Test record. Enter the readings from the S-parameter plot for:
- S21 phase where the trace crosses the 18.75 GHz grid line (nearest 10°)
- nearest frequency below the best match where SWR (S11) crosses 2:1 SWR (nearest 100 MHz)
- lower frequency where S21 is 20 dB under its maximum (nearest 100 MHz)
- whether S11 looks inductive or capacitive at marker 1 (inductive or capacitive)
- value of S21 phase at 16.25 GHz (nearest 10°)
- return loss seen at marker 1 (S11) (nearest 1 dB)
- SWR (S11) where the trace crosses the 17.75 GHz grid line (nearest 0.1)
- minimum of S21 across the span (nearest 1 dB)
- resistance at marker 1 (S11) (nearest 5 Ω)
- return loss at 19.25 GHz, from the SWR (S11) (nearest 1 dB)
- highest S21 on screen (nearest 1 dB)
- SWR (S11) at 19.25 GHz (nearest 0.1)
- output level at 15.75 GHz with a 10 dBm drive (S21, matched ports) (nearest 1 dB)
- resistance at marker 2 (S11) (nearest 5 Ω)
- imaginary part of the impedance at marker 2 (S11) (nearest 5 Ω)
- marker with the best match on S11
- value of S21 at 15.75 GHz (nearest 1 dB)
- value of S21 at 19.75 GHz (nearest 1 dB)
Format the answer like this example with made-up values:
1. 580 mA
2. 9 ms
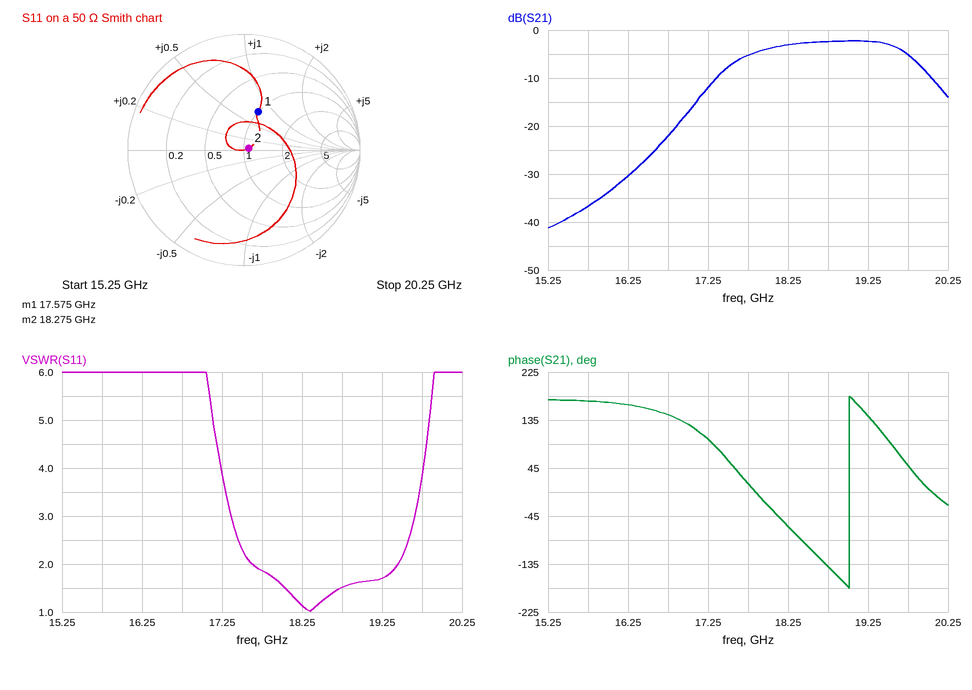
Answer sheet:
1. -140°
2. 17.6 GHz
3. 16.7 GHz
4. inductive
5. 160°
6. 9 dB
7. 1.9
8. -41 dB
9. 50 Ω
10. 12 dB
11. -2 dB
12. 1.7
13. -27 dBm
14. 55 Ω
15. 0 Ω
16. marker 2
17. -37 dB
18. -5 dB
